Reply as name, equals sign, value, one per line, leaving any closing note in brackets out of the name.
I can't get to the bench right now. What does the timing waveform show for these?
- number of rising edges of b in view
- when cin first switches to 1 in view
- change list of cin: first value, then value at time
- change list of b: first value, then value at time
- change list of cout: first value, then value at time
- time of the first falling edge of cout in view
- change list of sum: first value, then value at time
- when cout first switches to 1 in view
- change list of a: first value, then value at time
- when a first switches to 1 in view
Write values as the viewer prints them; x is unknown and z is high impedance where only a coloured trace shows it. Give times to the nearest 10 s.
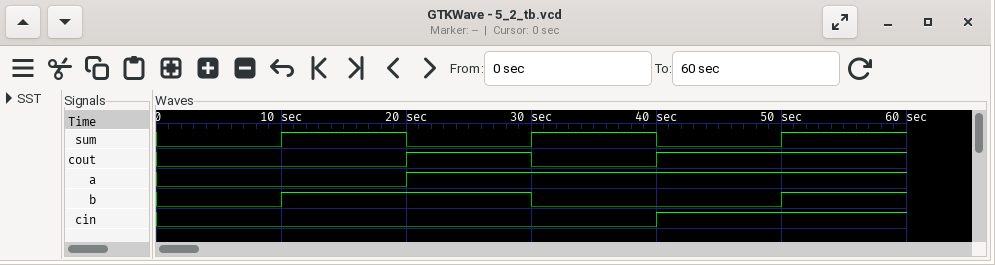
number of rising edges of b in view = 2
when cin first switches to 1 in view = 40 s
change list of cin: first value, then value at time = 0, 1 at 40 s
change list of b: first value, then value at time = 0, 1 at 10 s, 0 at 30 s, 1 at 50 s
change list of cout: first value, then value at time = 0, 1 at 20 s, 0 at 30 s, 1 at 40 s
time of the first falling edge of cout in view = 30 s
change list of sum: first value, then value at time = 0, 1 at 10 s, 0 at 20 s, 1 at 30 s, 0 at 40 s, 1 at 50 s
when cout first switches to 1 in view = 20 s
change list of a: first value, then value at time = 0, 1 at 20 s
when a first switches to 1 in view = 20 s
